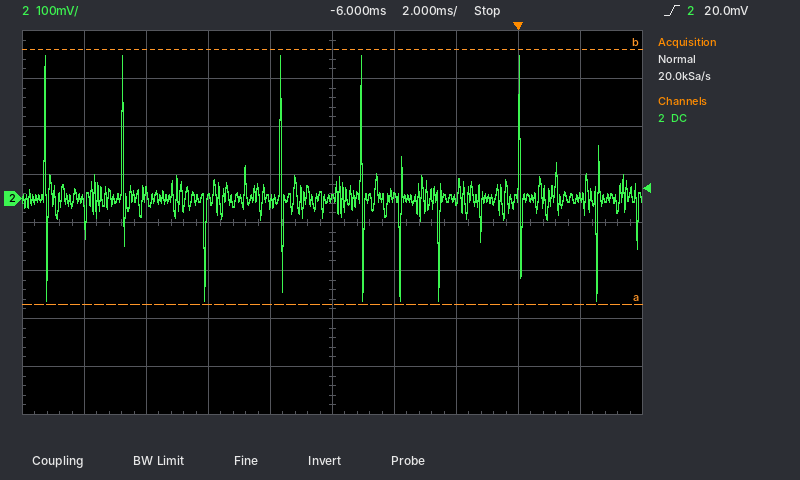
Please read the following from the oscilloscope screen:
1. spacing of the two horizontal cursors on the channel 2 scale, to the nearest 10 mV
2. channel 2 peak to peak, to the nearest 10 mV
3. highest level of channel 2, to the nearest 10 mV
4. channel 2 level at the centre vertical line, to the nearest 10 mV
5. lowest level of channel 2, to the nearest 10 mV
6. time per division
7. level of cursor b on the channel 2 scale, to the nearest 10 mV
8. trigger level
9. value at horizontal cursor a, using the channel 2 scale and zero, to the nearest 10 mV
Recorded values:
530 mV
510 mV
300 mV
0 mV
-210 mV
2 ms
310 mV
20.0 mV
-220 mV
